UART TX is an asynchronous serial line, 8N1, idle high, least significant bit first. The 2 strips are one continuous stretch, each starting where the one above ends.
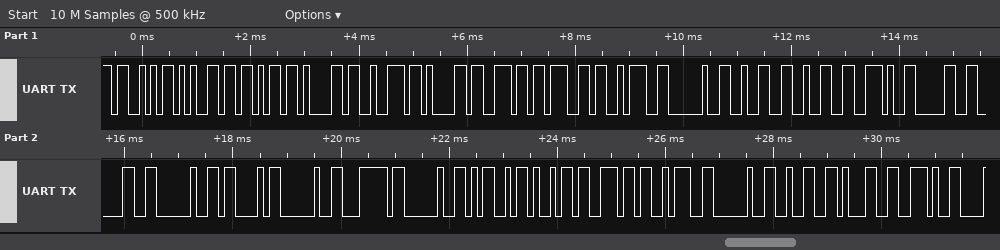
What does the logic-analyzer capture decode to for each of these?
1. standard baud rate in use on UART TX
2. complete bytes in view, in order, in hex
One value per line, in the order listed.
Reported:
9600 baud
53 65 6B 61 72 61 6E 67 3A 20 32 32 2E 30 30 20 43 20 7C 20 4D 69 6E 3A 20 32 31 2E
